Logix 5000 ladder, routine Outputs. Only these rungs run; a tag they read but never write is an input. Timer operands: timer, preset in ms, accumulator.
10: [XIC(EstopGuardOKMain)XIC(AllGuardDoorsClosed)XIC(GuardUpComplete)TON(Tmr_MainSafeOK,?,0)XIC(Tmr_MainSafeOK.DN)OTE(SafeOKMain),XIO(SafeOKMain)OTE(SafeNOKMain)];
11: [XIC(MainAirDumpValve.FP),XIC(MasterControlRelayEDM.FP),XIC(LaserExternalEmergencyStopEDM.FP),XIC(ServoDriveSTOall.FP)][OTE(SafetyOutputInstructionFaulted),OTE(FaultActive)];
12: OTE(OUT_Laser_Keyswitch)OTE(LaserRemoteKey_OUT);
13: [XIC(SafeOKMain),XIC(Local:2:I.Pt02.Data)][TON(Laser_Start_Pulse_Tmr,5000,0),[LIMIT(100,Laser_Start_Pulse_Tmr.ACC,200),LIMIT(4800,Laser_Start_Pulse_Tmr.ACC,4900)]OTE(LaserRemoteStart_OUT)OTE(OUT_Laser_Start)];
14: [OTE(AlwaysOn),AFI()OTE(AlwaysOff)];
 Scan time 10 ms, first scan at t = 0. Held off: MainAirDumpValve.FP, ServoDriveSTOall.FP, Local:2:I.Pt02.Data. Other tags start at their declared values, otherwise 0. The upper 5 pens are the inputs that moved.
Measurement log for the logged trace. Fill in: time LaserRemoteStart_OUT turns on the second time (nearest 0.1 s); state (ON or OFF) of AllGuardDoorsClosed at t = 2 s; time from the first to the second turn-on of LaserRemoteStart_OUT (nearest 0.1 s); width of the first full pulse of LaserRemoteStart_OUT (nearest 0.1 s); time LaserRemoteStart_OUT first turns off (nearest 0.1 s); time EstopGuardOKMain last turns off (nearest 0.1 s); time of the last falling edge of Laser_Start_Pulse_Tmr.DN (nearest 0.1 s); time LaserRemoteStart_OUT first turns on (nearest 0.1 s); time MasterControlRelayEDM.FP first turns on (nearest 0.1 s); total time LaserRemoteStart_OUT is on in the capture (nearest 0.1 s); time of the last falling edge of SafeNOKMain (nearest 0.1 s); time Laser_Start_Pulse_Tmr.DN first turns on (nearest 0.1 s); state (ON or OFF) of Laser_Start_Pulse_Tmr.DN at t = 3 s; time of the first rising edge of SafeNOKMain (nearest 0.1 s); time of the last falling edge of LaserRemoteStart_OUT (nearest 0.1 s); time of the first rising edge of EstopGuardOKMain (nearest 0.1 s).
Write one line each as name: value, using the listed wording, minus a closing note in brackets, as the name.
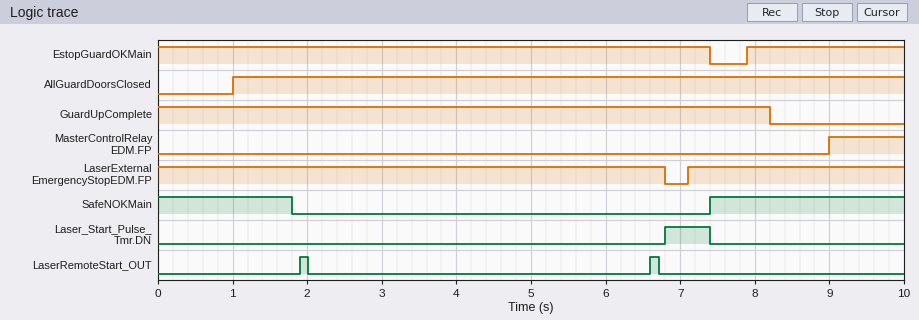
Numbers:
time LaserRemoteStart_OUT turns on the second time: 6.6 s
state (ON or OFF) of AllGuardDoorsClosed at t = 2 s: ON
time from the first to the second turn-on of LaserRemoteStart_OUT: 4.7 s
width of the first full pulse of LaserRemoteStart_OUT: 0.1 s
time LaserRemoteStart_OUT first turns off: 2.0 s
time EstopGuardOKMain last turns off: 7.4 s
time of the last falling edge of Laser_Start_Pulse_Tmr.DN: 7.4 s
time LaserRemoteStart_OUT first turns on: 1.9 s
time MasterControlRelayEDM.FP first turns on: 9.0 s
total time LaserRemoteStart_OUT is on in the capture: 0.2 s
time of the last falling edge of SafeNOKMain: 1.8 s
time Laser_Start_Pulse_Tmr.DN first turns on: 6.8 s
state (ON or OFF) of Laser_Start_Pulse_Tmr.DN at t = 3 s: OFF
time of the first rising edge of SafeNOKMain: 7.4 s
time of the last falling edge of LaserRemoteStart_OUT: 6.7 s
time of the first rising edge of EstopGuardOKMain: 7.9 s
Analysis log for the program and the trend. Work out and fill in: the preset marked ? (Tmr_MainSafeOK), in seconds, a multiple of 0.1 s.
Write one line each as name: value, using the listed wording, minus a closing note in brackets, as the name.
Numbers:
the preset marked ? (Tmr_MainSafeOK), in seconds, a multiple of 0.1 s: 0.8 s
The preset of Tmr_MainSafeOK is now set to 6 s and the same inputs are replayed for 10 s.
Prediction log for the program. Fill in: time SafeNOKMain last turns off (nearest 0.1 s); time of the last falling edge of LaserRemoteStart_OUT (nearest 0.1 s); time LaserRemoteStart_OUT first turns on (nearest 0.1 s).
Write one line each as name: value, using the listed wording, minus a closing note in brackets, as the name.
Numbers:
time SafeNOKMain last turns off: 7.0 s
time of the last falling edge of LaserRemoteStart_OUT: 7.2 s
time LaserRemoteStart_OUT first turns on: 7.1 s
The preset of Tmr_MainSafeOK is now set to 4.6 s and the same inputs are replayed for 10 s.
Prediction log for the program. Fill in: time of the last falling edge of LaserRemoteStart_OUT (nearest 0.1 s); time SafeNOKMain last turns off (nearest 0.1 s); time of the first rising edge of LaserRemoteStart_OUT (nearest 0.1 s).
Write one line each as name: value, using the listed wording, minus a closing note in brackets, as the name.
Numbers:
time of the last falling edge of LaserRemoteStart_OUT: 5.8 s
time SafeNOKMain last turns off: 5.6 s
time of the first rising edge of LaserRemoteStart_OUT: 5.7 s
